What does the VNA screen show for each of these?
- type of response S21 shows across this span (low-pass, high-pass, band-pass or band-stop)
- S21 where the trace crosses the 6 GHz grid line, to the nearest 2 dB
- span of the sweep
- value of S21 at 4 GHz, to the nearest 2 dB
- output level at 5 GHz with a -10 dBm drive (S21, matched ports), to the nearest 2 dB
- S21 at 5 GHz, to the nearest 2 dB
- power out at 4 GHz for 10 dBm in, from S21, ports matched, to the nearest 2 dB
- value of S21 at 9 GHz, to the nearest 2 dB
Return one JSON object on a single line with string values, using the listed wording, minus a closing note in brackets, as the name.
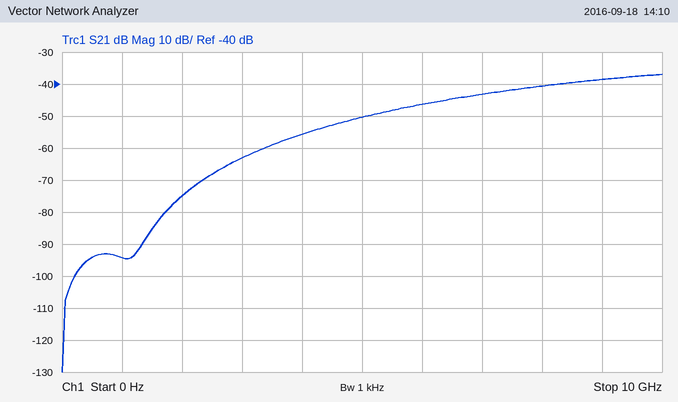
{"type of response S21 shows across this span": "high-pass", "S21 where the trace crosses the 6 GHz grid line, to the nearest 2 dB": "-46 dB", "span of the sweep": "10 GHz", "value of S21 at 4 GHz, to the nearest 2 dB": "-56 dB", "output level at 5 GHz with a -10 dBm drive (S21, matched ports), to the nearest 2 dB": "-60 dBm", "S21 at 5 GHz, to the nearest 2 dB": "-50 dB", "power out at 4 GHz for 10 dBm in, from S21, ports matched, to the nearest 2 dB": "-46 dBm", "value of S21 at 9 GHz, to the nearest 2 dB": "-38 dB"}
